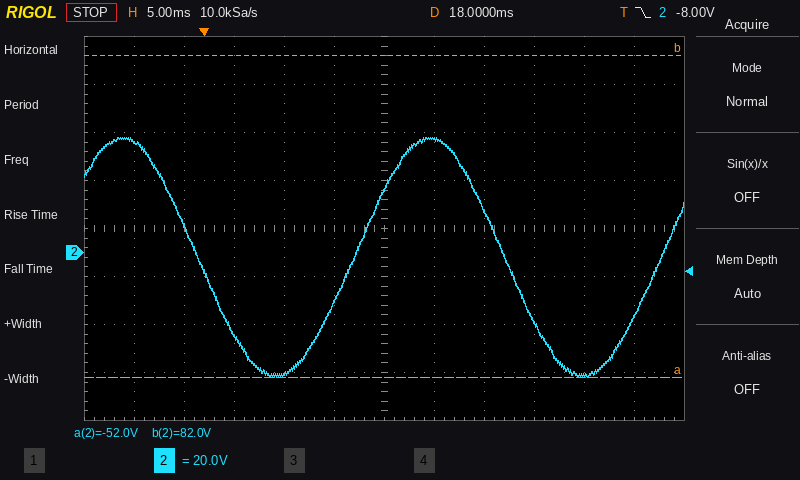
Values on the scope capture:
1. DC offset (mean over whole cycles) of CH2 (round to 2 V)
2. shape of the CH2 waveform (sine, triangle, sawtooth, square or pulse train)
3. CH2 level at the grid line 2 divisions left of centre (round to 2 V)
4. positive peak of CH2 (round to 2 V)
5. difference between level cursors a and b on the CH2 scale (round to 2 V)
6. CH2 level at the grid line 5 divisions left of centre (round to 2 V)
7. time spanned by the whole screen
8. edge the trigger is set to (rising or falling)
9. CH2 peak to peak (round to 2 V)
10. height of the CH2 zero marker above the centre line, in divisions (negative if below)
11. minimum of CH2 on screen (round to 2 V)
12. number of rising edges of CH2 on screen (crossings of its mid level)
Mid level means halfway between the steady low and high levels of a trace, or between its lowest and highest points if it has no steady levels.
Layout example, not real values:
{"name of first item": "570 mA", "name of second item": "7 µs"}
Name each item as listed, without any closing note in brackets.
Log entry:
{"DC offset (mean over whole cycles) of CH2": "-2 V", "shape of the CH2 waveform": "sine", "CH2 level at the grid line 2 divisions left of centre": "-50 V", "positive peak of CH2": "48 V", "difference between level cursors a and b on the CH2 scale": "134 V", "CH2 level at the grid line 5 divisions left of centre": "46 V", "time spanned by the whole screen": "60 ms", "edge the trigger is set to": "falling", "CH2 peak to peak": "100 V", "height of the CH2 zero marker above the centre line, in divisions": "-0.5 div", "minimum of CH2 on screen": "-52 V", "number of rising edges of CH2 on screen": "2"}
